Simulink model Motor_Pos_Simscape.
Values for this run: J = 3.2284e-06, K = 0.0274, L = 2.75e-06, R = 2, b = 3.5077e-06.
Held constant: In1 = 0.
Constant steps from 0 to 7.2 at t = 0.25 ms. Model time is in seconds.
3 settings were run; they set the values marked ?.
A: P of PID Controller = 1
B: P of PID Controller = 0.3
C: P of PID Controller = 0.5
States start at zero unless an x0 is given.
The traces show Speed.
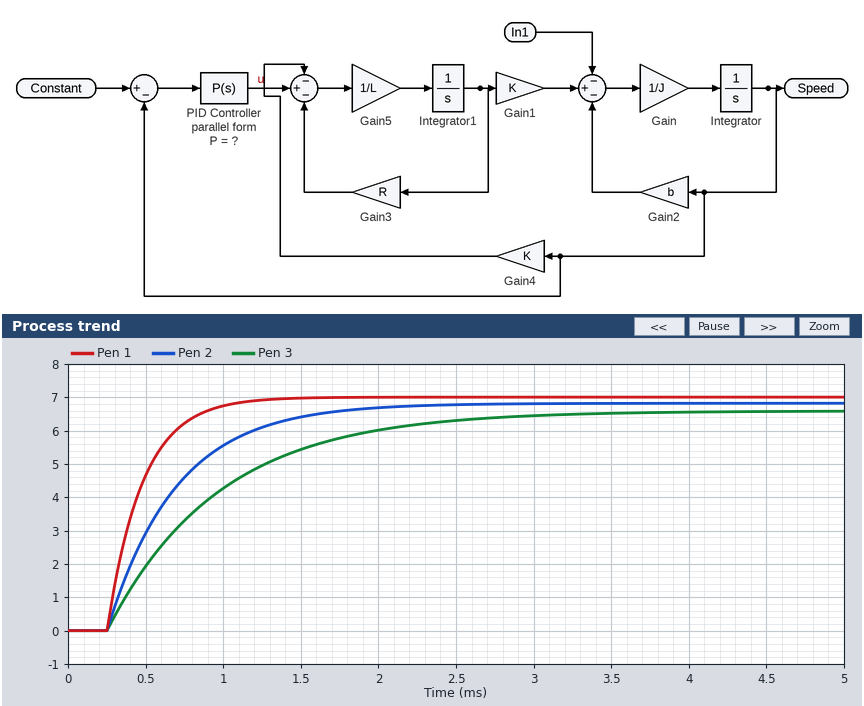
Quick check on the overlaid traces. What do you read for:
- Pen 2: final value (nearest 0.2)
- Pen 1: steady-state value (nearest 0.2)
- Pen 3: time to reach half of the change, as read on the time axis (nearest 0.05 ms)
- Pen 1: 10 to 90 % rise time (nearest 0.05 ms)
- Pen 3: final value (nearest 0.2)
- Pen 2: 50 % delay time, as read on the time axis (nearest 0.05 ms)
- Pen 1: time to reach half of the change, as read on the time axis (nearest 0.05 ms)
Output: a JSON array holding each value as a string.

["6.8", "7.0", "0.75 ms", "0.50 ms", "6.6", "0.55 ms", "0.40 ms"]
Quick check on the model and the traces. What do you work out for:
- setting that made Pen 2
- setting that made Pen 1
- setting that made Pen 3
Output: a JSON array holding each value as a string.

["C", "A", "B"]
